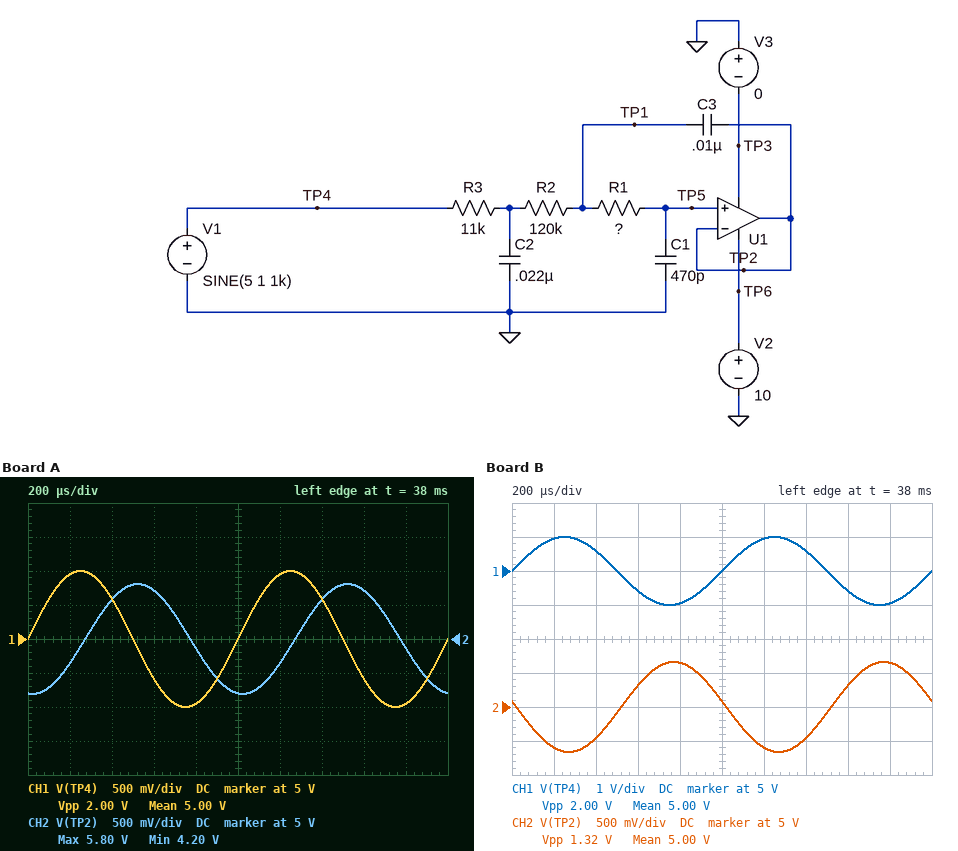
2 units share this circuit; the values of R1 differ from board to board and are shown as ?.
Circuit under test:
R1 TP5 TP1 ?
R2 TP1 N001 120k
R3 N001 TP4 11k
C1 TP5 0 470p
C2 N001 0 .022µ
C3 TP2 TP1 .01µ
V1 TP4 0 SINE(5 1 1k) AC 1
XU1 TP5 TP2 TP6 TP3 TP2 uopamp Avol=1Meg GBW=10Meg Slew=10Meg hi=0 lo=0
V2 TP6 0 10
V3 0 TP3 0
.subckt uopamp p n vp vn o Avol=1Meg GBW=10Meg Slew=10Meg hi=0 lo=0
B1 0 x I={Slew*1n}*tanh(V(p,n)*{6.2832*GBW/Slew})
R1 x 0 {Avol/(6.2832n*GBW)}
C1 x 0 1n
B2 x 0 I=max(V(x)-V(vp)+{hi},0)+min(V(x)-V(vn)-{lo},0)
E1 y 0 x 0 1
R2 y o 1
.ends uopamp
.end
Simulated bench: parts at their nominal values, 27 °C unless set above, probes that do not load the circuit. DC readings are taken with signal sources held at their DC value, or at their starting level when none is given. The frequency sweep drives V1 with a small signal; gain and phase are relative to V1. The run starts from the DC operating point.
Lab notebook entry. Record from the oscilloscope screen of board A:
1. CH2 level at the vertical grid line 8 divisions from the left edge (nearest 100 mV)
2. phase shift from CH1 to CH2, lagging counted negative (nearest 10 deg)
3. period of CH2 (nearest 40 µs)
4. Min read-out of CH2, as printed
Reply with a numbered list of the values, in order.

1. 5.7 V
2. -100 deg
3. 1.00 ms
4. 4.20 V
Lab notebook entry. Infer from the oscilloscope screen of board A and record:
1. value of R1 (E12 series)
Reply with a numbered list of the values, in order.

1. 22 kΩ
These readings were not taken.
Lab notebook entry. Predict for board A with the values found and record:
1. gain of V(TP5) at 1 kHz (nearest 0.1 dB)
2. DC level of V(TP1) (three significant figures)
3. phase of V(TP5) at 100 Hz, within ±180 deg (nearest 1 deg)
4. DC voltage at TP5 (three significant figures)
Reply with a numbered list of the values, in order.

1. -1.9 dB
2. 5.00 V
3. -11 deg
4. 5.00 V
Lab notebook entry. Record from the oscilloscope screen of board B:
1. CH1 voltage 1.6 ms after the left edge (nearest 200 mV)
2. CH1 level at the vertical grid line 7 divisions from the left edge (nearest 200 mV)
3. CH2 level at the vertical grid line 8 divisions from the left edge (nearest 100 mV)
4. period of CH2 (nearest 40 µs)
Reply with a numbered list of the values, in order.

1. 4.4 V
2. 5.6 V
3. 5.3 V
4. 1.00 ms
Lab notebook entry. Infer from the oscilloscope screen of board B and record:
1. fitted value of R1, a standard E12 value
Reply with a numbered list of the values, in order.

1. 68 kΩ
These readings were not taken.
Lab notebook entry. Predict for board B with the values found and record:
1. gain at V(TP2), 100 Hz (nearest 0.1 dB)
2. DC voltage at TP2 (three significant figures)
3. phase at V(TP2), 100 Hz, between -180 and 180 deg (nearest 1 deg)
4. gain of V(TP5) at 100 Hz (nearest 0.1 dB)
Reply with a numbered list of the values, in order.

1. 0 dB
2. 5.00 V
3. -12 deg
4. 0 dB
